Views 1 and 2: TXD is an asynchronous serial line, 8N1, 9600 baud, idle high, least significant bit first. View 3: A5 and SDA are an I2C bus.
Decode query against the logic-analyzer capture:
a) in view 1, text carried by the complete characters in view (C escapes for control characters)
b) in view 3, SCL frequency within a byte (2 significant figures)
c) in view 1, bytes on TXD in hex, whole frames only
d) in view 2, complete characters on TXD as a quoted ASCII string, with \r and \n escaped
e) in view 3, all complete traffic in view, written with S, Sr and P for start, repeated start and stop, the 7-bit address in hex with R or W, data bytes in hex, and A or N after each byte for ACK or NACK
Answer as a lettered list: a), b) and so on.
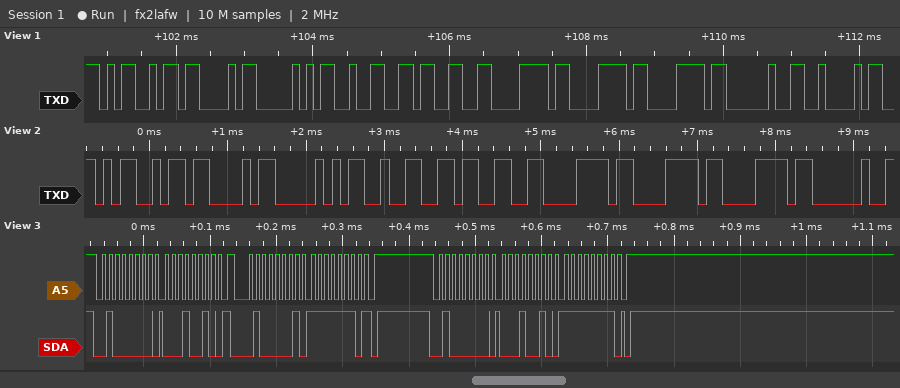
a) "MCP23xxx B"
b) 100 kHz
c) 4D 43 50 32 33 78 78 78 20 42
d) "MCP23xxx "
e) S 20W A 12 A Sr 20R A FE N P S 20W A 12 A FF A P
